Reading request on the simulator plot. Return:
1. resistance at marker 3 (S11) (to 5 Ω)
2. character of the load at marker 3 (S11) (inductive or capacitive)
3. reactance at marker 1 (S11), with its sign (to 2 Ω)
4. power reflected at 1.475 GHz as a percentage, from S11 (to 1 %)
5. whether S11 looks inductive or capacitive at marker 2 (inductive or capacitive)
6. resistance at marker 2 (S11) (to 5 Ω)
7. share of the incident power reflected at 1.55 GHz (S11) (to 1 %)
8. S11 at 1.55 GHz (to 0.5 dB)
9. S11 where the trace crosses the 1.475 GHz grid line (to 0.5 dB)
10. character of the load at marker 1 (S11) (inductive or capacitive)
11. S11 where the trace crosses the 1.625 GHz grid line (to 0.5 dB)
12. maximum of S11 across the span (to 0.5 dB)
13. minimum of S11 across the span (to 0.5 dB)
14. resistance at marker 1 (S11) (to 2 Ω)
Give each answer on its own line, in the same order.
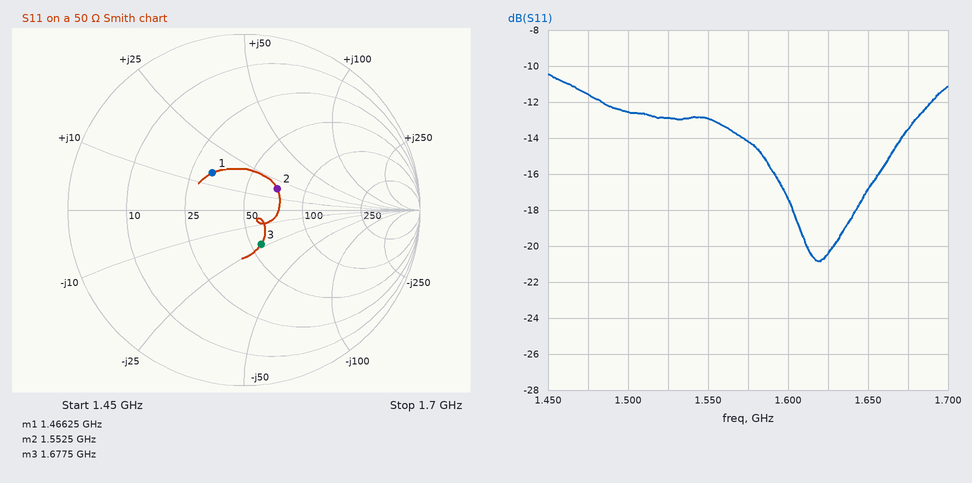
55 Ω
capacitive
+14 Ω
7 %
inductive
70 Ω
5 %
-13.0 dB
-11.5 dB
inductive
-20.5 dB
-10.5 dB
-21.0 dB
32 Ω
